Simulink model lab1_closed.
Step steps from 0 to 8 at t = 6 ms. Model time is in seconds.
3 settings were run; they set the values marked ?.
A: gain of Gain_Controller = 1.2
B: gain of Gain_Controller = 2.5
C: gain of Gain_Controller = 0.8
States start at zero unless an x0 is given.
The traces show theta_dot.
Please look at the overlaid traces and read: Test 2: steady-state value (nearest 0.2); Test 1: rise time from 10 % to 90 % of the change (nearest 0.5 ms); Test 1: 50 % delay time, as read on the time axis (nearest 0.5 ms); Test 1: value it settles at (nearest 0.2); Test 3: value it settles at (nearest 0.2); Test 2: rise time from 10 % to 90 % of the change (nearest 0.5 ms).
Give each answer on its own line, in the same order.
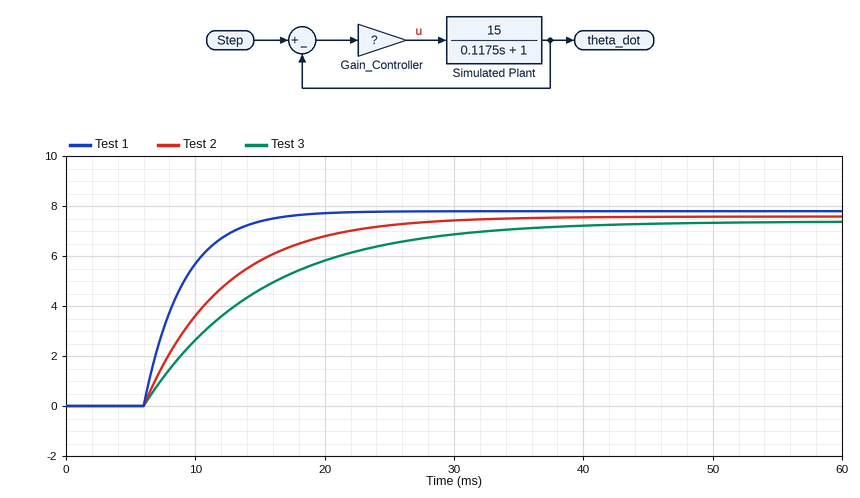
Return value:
7.6
6.5 ms
8.0 ms
7.8
7.4
13.5 ms
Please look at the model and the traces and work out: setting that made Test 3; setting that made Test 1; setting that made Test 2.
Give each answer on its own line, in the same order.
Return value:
C
B
A
